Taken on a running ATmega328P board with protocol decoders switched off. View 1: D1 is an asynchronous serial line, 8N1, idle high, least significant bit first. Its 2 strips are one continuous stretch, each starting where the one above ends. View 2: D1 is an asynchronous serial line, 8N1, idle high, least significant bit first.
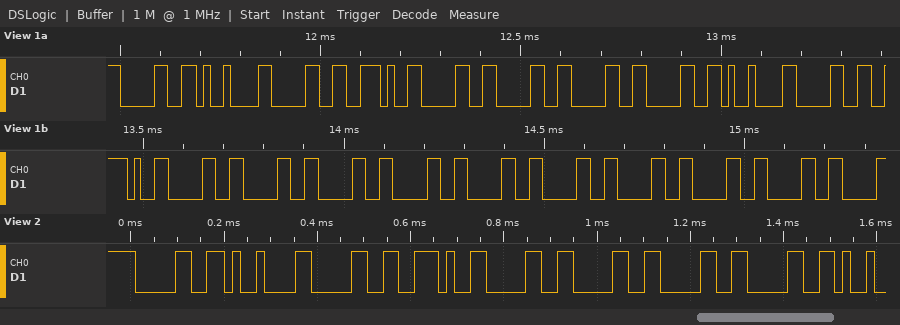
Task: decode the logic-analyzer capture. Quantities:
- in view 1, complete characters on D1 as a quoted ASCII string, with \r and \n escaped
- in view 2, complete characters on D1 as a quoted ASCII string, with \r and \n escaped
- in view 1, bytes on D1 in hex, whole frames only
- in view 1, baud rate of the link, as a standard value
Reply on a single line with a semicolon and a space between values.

"0\t0.0000\t0.000000000"; "0\t0.0000"; 0x30 0x09 0x30 0x2E 0x30 0x30 0x30 0x30 0x09 0x30 0x2E 0x30 0x30 0x30 0x30 0x30 0x30 0x30 0x30 0x30; 57600 baud
